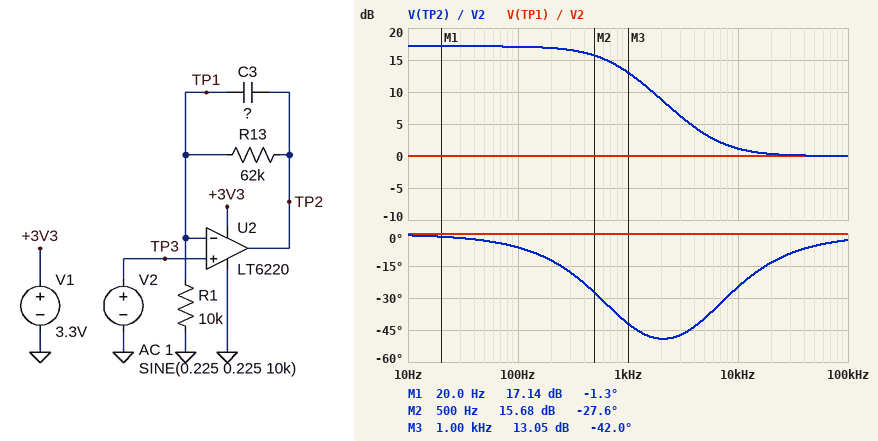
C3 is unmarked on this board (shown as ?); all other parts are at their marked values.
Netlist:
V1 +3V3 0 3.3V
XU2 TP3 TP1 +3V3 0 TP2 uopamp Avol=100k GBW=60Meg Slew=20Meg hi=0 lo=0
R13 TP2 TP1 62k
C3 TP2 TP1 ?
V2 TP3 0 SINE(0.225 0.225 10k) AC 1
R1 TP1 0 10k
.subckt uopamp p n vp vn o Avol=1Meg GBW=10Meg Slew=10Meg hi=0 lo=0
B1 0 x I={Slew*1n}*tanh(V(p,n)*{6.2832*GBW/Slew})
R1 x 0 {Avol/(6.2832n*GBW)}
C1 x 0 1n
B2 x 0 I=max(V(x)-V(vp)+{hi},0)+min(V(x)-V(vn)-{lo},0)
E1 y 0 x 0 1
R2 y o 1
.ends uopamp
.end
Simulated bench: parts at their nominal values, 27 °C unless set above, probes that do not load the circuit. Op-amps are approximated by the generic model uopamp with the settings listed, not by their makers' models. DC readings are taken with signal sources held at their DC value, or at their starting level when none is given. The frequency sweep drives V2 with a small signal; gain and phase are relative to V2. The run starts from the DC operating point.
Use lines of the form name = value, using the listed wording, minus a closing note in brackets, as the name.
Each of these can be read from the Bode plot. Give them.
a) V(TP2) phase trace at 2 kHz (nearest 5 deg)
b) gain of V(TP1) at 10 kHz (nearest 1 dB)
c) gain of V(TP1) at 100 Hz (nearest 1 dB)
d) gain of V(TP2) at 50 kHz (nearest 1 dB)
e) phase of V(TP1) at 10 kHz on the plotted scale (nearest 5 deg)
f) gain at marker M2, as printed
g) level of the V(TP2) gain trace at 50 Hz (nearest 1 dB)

V(TP2) phase trace at 2 kHz = -50 deg
gain of V(TP1) at 10 kHz = 0 dB
gain of V(TP1) at 100 Hz = 0 dB
gain of V(TP2) at 50 kHz = 0 dB
phase of V(TP1) at 10 kHz on the plotted scale = 0 deg
gain at marker M2, as printed = 15.68 dB
level of the V(TP2) gain trace at 50 Hz = 17 dB
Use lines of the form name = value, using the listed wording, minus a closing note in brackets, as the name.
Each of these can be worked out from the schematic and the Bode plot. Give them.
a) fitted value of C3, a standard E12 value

fitted value of C3, a standard E12 value = 3.3 nF
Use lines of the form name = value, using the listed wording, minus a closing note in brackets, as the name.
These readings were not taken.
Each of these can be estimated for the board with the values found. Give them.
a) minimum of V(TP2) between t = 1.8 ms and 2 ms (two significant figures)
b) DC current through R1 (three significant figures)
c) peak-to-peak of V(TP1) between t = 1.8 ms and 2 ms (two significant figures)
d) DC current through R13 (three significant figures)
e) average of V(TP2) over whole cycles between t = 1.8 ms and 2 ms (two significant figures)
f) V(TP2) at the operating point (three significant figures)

minimum of V(TP2) between t = 1.8 ms and 2 ms = 1.4 V
DC current through R1 = 22.5 µA
peak-to-peak of V(TP1) between t = 1.8 ms and 2 ms = 450 mV
DC current through R13 = 22.5 µA
average of V(TP2) over whole cycles between t = 1.8 ms and 2 ms = 1.6 V
V(TP2) at the operating point = 1.62 V
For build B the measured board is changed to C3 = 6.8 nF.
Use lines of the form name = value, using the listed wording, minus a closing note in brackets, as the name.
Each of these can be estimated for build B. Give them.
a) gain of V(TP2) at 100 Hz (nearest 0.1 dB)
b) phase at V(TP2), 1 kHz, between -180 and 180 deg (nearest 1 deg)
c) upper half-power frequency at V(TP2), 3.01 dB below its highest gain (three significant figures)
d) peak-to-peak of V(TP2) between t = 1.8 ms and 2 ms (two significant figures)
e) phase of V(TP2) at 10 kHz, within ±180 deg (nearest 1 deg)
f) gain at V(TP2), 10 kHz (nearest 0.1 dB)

gain of V(TP2) at 100 Hz = 16.9 dB
phase at V(TP2), 1 kHz, between -180 and 180 deg = -49 deg
upper half-power frequency at V(TP2), 3.01 dB below its highest gain = 385 Hz
peak-to-peak of V(TP2) between t = 1.8 ms and 2 ms = 470 mV
phase of V(TP2) at 10 kHz, within ±180 deg = -13 deg
gain at V(TP2), 10 kHz = 0.3 dB
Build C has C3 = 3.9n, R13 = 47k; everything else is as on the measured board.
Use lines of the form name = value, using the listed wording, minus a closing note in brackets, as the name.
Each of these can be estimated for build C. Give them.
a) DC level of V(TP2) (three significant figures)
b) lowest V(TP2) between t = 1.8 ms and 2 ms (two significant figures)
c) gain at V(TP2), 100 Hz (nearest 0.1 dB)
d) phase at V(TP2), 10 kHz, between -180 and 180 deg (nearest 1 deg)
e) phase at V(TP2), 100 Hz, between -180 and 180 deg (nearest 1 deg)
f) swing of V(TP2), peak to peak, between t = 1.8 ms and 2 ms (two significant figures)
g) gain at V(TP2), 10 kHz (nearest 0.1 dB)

DC level of V(TP2) = 1.28 V
lowest V(TP2) between t = 1.8 ms and 2 ms = 1.0 V
gain at V(TP2), 100 Hz = 15.1 dB
phase at V(TP2), 10 kHz, between -180 and 180 deg = -21 deg
phase at V(TP2), 100 Hz, between -180 and 180 deg = -5 deg
swing of V(TP2), peak to peak, between t = 1.8 ms and 2 ms = 500 mV
gain at V(TP2), 10 kHz = 0.9 dB
